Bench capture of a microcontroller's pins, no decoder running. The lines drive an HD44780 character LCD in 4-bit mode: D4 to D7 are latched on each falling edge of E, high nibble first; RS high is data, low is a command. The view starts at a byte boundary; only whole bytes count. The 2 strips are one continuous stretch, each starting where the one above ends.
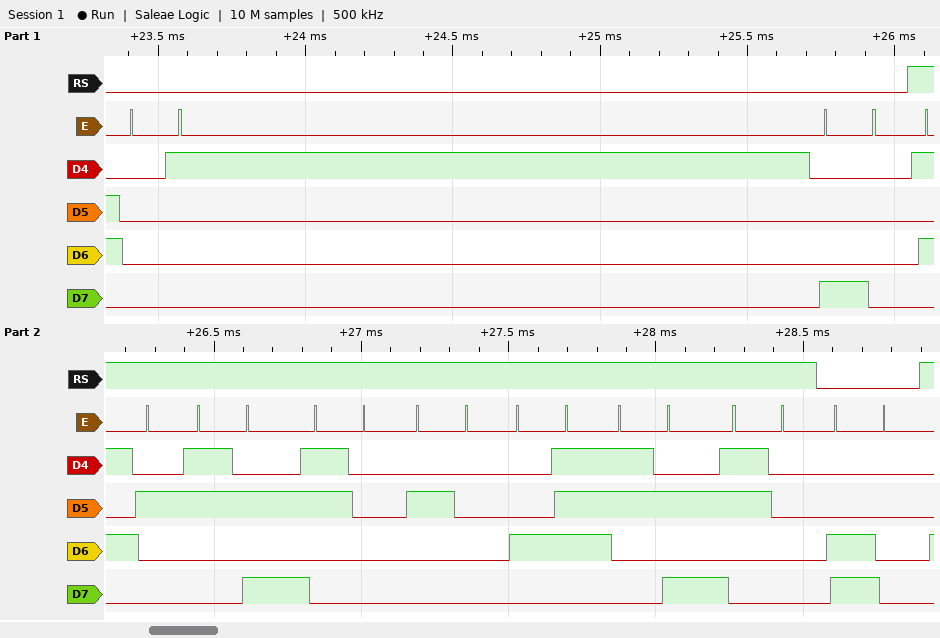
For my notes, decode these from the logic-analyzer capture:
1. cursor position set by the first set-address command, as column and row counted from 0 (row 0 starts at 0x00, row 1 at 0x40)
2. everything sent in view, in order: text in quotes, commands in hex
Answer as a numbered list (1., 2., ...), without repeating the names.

1. column 0, row 0
2. 0x01 0x80 "R:0 G:0" 0xC0
